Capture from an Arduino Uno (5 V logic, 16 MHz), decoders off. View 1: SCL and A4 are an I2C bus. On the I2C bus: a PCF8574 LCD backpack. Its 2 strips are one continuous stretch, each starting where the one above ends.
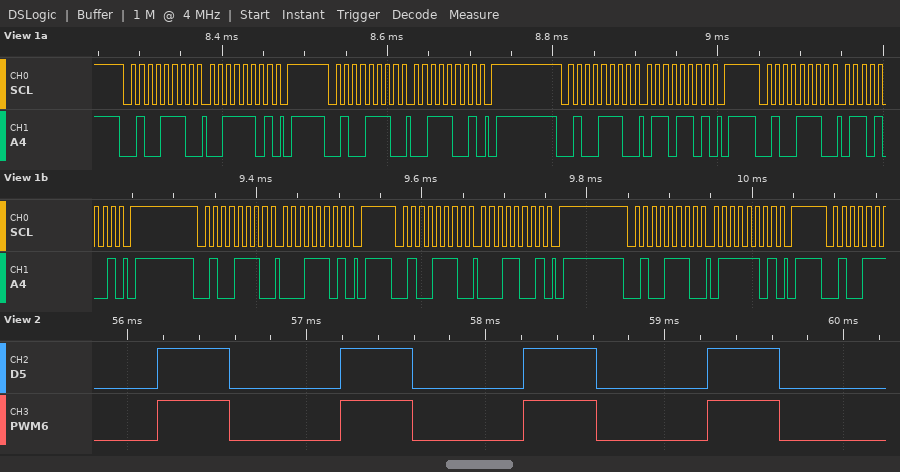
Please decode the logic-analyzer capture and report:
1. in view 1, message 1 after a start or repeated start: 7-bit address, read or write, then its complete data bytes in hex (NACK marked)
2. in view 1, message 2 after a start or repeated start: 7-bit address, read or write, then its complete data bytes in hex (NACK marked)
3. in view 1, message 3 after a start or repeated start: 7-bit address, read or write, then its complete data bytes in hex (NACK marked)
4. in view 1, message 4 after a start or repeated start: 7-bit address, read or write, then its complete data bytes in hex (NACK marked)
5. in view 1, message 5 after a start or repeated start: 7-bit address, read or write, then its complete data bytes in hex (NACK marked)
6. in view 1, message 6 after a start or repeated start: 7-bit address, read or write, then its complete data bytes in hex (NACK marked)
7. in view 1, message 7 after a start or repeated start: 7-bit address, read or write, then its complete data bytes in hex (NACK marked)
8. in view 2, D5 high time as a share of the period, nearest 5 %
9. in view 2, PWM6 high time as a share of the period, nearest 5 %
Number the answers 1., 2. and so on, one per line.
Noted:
1. 0x27 write: 3D
2. 0x27 write: 39
3. 0x27 write: 6D
4. 0x27 write: 69
5. 0x27 write: 1D
6. 0x27 write: 19
7. 0x27 write: 7D
8. 40 %
9. 40 %
